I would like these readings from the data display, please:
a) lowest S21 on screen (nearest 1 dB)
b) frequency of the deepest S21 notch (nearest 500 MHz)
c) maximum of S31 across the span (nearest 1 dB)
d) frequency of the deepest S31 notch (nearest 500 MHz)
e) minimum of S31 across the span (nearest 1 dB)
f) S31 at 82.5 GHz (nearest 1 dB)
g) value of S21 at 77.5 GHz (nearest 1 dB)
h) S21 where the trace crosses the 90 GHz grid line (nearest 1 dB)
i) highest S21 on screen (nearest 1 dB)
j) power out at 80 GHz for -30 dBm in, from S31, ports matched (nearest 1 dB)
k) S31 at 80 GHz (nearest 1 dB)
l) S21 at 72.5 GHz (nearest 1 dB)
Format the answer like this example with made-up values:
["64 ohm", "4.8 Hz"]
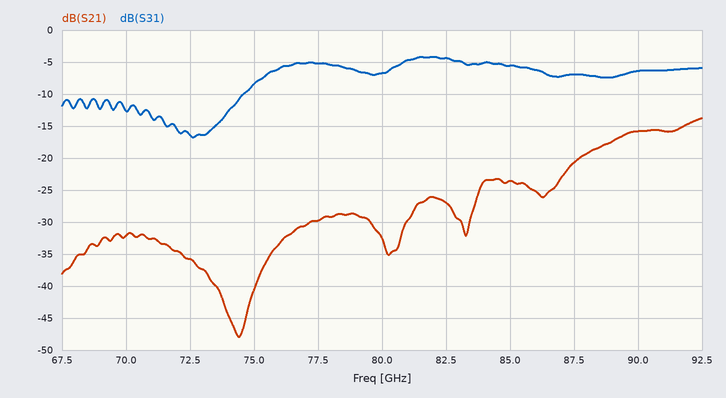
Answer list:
["-48 dB", "74.5 GHz", "-4 dB", "72.5 GHz", "-17 dB", "-4 dB", "-30 dB", "-16 dB", "-14 dB", "-37 dBm", "-7 dB", "-36 dB"]
